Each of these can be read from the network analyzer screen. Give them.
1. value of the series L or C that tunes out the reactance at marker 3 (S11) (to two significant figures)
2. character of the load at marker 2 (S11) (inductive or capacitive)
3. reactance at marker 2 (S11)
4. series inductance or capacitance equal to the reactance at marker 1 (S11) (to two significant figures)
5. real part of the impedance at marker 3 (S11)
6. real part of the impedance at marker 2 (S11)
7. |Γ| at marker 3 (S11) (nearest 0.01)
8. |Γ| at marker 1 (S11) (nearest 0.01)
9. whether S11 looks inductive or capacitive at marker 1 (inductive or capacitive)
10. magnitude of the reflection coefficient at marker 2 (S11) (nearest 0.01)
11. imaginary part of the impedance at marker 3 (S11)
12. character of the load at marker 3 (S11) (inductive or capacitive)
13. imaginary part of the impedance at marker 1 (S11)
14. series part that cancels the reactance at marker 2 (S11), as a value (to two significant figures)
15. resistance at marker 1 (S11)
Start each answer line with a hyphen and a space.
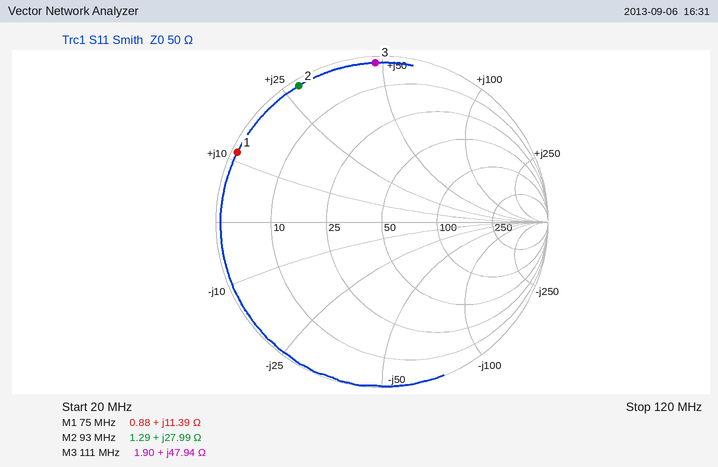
- 30 pF
- inductive
- +27.99 Ω
- 24 nH
- 1.90 Ω
- 1.29 Ω
- 0.96
- 0.97
- inductive
- 0.96
- +47.94 Ω
- inductive
- +11.39 Ω
- 61 pF
- 0.88 Ω
